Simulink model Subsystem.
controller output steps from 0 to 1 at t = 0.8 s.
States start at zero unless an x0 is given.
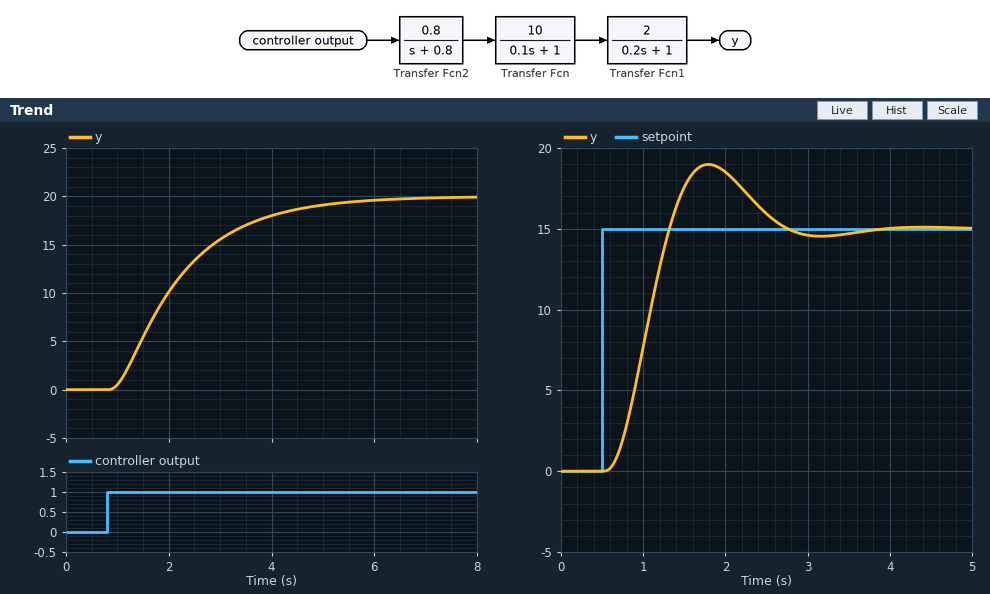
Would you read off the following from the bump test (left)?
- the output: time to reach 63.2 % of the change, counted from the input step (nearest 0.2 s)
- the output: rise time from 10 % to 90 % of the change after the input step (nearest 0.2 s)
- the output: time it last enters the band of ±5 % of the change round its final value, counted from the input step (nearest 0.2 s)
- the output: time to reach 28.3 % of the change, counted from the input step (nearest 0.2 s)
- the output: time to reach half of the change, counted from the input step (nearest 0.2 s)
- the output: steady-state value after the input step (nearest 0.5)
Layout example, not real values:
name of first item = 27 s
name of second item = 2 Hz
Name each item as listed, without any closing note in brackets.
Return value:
the output: time to reach 63.2 % of the change, counted from the input step = 1.6 s
the output: rise time from 10 % to 90 % of the change after the input step = 2.8 s
the output: time it last enters the band of ±5 % of the change round its final value, counted from the input step = 4.0 s
the output: time to reach 28.3 % of the change, counted from the input step = 0.8 s
the output: time to reach half of the change, counted from the input step = 1.2 s
the output: steady-state value after the input step = 20.0
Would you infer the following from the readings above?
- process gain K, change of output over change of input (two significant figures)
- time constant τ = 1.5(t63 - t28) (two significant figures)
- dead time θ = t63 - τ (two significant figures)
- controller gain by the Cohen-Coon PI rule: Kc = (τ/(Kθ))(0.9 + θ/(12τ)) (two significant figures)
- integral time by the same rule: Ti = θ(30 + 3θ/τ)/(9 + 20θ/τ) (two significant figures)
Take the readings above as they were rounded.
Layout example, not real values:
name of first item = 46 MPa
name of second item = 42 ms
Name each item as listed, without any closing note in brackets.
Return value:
process gain K, change of output over change of input = 20
time constant τ = 1.5(t63 - t28) = 1.2 s
dead time θ = t63 - τ = 0.40 s
controller gain by the Cohen-Coon PI rule: Kc = (τ/(Kθ))(0.9 + θ/(12τ)) = 0.14
integral time by the same rule: Ti = θ(30 + 3θ/τ)/(9 + 20θ/τ) = 0.79 s
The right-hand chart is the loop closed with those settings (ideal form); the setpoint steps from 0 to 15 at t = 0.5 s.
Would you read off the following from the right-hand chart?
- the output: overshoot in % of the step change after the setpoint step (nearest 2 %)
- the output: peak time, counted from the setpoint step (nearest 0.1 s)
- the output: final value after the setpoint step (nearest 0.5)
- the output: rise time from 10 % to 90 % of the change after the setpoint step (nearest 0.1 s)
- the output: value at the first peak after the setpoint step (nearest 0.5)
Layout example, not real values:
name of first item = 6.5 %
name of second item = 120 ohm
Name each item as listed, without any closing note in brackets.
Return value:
the output: overshoot in % of the step change after the setpoint step = 26 %
the output: peak time, counted from the setpoint step = 1.3 s
the output: final value after the setpoint step = 15.0
the output: rise time from 10 % to 90 % of the change after the setpoint step = 0.5 s
the output: value at the first peak after the setpoint step = 19.0
